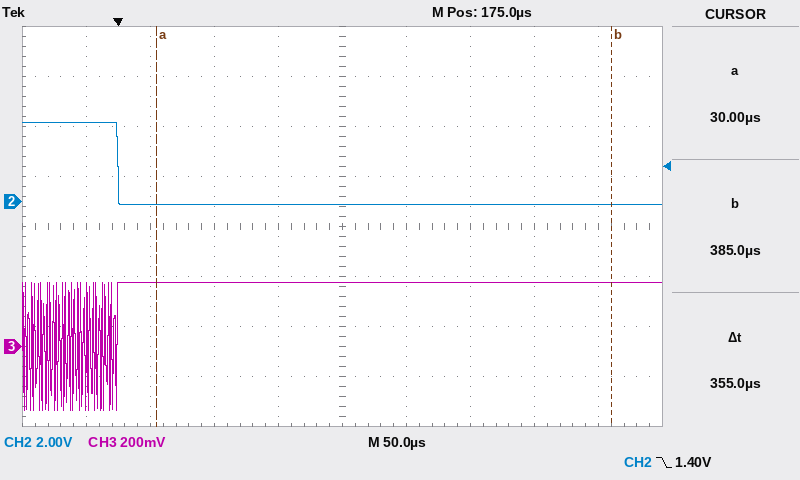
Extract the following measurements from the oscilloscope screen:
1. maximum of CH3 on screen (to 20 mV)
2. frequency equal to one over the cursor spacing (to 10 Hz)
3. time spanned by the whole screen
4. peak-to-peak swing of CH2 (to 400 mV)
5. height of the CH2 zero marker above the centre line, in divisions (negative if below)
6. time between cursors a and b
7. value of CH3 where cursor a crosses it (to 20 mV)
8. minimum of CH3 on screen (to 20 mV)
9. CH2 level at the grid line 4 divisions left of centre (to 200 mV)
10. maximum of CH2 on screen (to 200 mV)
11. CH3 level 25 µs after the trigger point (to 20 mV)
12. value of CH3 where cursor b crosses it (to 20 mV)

260 mV
2.82 kHz
500 µs
3.2 V
+0.5 div
355 µs
260 mV
-260 mV
3.2 V
3.2 V
260 mV
260 mV
